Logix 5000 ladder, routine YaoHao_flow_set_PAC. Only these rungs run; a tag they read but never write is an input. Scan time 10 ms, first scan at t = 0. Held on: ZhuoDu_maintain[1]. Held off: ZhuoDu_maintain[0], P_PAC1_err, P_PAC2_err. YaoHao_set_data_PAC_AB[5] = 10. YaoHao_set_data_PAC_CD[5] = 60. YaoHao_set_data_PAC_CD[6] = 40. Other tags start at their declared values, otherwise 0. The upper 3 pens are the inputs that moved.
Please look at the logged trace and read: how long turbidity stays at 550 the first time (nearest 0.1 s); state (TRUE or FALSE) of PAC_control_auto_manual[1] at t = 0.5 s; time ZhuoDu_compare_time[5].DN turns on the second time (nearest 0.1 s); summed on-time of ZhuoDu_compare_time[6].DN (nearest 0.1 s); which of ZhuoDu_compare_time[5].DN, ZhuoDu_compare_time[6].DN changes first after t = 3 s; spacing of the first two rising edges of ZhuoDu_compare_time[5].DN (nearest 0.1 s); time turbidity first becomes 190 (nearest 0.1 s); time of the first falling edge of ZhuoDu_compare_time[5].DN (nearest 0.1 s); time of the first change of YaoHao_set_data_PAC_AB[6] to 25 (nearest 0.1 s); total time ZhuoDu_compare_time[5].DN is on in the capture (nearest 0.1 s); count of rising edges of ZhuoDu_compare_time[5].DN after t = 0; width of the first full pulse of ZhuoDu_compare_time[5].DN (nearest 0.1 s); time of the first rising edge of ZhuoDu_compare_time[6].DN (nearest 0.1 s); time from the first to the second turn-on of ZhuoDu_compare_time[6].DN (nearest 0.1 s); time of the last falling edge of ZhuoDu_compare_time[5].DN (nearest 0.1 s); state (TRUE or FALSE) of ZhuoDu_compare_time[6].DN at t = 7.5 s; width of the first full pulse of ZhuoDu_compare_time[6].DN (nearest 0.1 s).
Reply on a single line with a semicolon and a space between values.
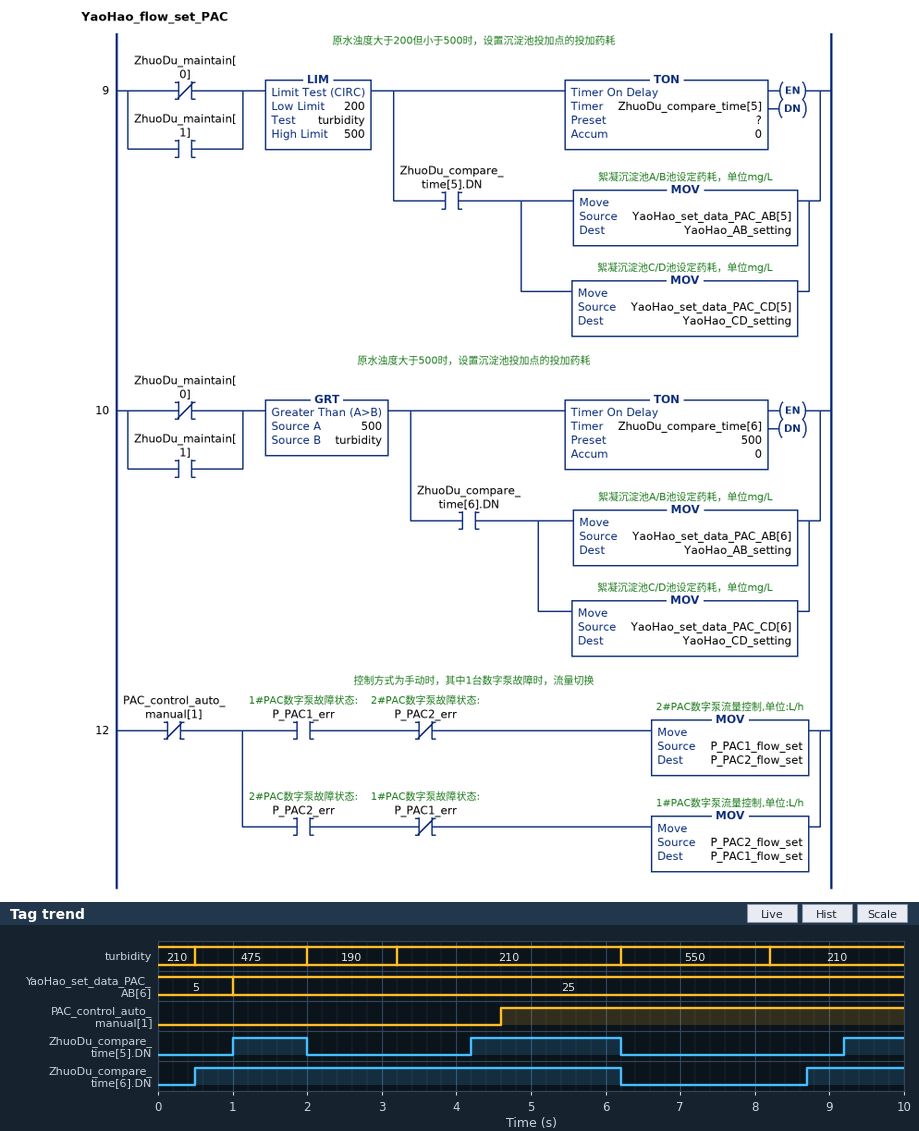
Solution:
2.0 s; FALSE; 4.2 s; 7.0 s; ZhuoDu_compare_time[5].DN; 3.2 s; 2.0 s; 2.0 s; 1.0 s; 3.8 s; 3; 1.0 s; 0.5 s; 8.2 s; 6.2 s; FALSE; 5.7 s
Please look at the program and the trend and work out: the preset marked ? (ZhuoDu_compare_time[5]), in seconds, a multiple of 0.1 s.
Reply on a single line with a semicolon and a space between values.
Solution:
1.0 s
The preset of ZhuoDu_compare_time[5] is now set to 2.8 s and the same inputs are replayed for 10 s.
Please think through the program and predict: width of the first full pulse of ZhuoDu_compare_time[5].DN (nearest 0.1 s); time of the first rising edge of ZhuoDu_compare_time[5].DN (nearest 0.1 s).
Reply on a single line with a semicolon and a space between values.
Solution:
0.2 s; 6.0 s
